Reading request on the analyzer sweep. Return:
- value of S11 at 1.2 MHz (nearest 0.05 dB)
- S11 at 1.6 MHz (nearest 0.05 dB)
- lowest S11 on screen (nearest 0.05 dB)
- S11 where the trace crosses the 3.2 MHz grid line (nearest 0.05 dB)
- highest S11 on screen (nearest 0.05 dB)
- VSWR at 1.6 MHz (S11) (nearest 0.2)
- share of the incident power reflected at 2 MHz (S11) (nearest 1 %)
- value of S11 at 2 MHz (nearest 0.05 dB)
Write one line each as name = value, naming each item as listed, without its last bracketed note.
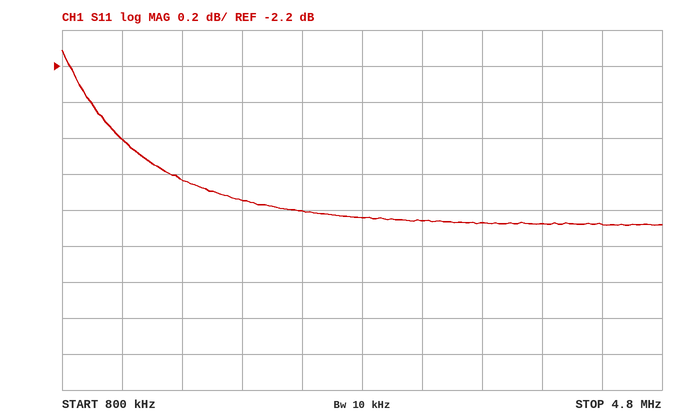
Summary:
value of S11 at 1.2 MHz = -2.60 dB
S11 at 1.6 MHz = -2.85 dB
lowest S11 on screen = -3.10 dB
S11 where the trace crosses the 3.2 MHz grid line = -3.05 dB
highest S11 on screen = -2.10 dB
VSWR at 1.6 MHz (S11) = 6.2
share of the incident power reflected at 2 MHz (S11) = 51 %
value of S11 at 2 MHz = -2.95 dB
